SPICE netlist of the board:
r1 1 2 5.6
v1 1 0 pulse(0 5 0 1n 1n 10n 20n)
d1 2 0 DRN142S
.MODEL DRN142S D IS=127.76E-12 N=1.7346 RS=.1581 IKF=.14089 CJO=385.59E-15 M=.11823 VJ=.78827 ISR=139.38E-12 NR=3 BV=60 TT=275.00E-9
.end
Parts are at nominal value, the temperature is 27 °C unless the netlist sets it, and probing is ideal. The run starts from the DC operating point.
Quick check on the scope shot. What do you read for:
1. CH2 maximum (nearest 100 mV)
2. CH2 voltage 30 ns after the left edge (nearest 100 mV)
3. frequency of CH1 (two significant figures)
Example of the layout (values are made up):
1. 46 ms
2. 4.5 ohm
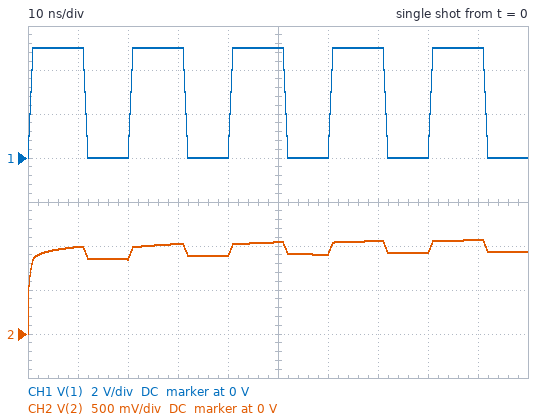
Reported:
1. 1.1 V
2. 1.0 V
3. 50 MHz
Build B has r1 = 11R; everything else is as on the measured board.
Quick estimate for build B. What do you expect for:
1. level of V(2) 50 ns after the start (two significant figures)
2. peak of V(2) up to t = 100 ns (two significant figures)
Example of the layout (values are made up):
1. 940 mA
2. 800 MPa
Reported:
1. 950 mV
2. 980 mV
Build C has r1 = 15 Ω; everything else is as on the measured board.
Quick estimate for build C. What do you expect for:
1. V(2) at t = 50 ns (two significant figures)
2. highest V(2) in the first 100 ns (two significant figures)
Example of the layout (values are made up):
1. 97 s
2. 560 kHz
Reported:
1. 920 mV
2. 940 mV
